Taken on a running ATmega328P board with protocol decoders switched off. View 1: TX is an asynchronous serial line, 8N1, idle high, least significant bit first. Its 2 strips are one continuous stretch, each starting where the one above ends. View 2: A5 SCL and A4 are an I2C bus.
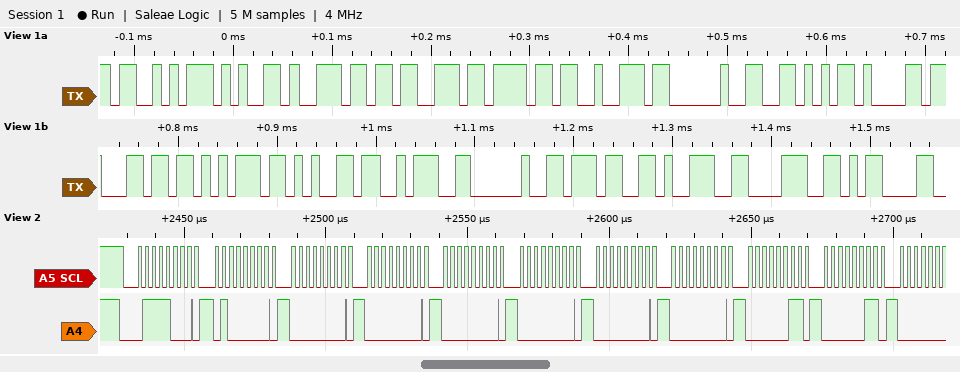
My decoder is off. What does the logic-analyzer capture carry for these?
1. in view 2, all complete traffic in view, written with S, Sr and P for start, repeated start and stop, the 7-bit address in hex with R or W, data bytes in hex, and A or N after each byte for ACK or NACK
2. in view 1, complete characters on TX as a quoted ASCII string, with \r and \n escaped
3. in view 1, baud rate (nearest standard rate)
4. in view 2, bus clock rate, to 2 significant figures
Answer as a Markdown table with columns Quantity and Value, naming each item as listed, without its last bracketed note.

| Quantity | Value |
|---|---|
| in view 2, all complete traffic in view, written with S, Sr and P for start, repeated start and stop, the 7-bit address in hex with R or W, data bytes in hex, and A or N after each byte for ACK or NACK | S 3CW A 40 A 00 A 00 A 00 A 00 A 00 A 00 A 03 A 03 A |
| in view 1, complete characters on TX as a quoted ASCII string, with \r and \n escaped | "Sensor Value: 798\r" |
| in view 1, baud rate | 115200 baud |
| in view 2, bus clock rate, to 2 significant figures | 400 kHz |
